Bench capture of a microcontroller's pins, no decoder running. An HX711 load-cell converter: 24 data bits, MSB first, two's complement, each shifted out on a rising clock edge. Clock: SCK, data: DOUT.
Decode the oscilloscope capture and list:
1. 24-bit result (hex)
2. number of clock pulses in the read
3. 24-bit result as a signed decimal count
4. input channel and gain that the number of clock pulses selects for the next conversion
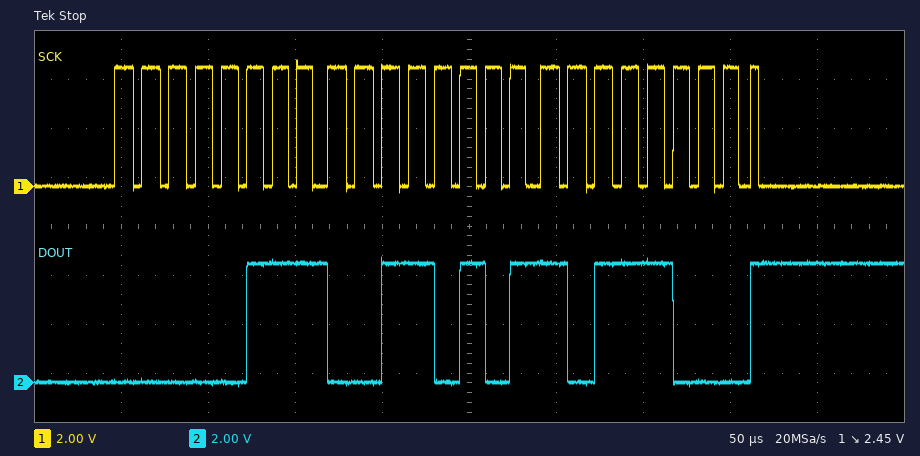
0x0735B8
25
472504
channel A, gain 128
